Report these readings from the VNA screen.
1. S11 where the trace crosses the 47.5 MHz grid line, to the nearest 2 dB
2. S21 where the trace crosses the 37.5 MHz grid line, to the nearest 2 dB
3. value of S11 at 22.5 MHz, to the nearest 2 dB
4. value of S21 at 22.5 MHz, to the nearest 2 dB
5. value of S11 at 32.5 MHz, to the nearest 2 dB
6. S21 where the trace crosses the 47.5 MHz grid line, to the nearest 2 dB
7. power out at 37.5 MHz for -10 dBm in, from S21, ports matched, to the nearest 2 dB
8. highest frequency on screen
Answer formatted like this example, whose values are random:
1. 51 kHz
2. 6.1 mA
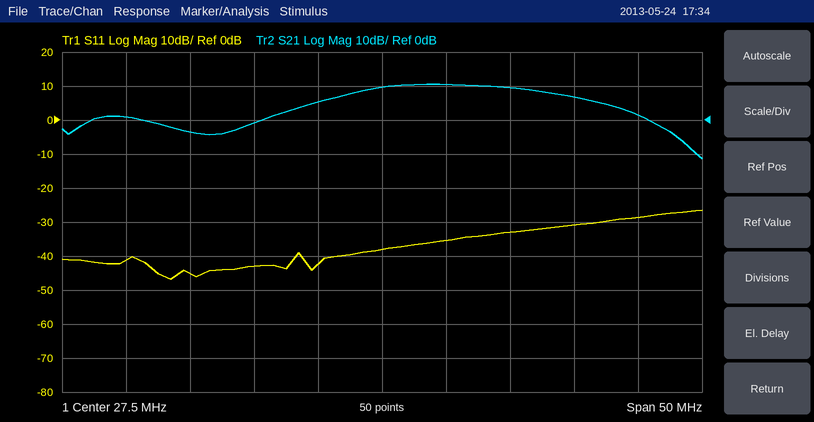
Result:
1. -28 dB
2. 10 dB
3. -42 dB
4. 6 dB
5. -36 dB
6. 2 dB
7. 0 dBm
8. 52.5 MHz
